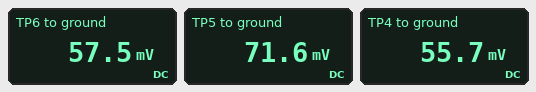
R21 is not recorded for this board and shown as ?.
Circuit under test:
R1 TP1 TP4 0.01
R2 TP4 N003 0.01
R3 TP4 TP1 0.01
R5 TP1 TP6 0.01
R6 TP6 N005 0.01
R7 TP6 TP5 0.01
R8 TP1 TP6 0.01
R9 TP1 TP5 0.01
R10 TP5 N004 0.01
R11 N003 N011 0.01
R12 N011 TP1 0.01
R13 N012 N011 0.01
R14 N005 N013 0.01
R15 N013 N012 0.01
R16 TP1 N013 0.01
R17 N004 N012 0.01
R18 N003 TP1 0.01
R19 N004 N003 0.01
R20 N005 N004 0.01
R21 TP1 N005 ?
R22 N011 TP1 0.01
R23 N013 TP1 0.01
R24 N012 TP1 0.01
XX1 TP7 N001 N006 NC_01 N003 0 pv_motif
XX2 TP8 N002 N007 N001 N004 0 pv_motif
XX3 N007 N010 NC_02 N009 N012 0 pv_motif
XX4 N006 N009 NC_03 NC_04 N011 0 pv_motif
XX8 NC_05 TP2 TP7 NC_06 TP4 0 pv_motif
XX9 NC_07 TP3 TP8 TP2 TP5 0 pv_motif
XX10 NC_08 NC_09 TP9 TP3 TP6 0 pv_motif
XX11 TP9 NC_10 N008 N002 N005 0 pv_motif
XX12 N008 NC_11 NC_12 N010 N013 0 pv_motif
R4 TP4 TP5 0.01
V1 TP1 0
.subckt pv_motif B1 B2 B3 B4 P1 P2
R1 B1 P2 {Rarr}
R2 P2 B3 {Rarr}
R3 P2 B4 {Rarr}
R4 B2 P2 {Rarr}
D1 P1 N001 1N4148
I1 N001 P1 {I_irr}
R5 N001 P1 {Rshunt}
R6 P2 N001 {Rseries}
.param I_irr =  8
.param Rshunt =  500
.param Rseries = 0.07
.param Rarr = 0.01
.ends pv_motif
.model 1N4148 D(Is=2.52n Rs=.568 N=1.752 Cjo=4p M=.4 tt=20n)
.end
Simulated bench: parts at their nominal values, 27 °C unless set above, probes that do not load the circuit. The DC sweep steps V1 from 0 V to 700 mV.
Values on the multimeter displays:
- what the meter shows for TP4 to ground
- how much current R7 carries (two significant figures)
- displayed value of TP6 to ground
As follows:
55.7 mV
1.4 A
57.5 mV
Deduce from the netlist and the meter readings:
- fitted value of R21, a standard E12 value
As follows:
0.015 Ω
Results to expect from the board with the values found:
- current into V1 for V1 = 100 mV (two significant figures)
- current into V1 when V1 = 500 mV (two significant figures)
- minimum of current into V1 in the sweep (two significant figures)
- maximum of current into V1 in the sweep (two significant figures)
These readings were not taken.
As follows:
72 A
68 A
66 A
72 A
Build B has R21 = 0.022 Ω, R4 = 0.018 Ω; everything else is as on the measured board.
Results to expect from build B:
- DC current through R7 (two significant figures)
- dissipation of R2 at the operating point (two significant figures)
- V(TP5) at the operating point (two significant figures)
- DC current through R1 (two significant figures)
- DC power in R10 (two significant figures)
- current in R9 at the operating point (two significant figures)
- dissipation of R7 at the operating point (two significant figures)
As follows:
1.5 A
30 mW
75 mV
5.4 A
46 mW
7.5 A
22 mW
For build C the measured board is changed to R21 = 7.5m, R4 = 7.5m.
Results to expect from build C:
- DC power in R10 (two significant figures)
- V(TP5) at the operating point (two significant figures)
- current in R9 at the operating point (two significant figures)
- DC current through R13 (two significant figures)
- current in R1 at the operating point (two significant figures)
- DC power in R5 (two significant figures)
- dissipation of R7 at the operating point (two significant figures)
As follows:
38 mW
68 mV
6.8 A
1.4 A
5.5 A
280 mW
23 mW
